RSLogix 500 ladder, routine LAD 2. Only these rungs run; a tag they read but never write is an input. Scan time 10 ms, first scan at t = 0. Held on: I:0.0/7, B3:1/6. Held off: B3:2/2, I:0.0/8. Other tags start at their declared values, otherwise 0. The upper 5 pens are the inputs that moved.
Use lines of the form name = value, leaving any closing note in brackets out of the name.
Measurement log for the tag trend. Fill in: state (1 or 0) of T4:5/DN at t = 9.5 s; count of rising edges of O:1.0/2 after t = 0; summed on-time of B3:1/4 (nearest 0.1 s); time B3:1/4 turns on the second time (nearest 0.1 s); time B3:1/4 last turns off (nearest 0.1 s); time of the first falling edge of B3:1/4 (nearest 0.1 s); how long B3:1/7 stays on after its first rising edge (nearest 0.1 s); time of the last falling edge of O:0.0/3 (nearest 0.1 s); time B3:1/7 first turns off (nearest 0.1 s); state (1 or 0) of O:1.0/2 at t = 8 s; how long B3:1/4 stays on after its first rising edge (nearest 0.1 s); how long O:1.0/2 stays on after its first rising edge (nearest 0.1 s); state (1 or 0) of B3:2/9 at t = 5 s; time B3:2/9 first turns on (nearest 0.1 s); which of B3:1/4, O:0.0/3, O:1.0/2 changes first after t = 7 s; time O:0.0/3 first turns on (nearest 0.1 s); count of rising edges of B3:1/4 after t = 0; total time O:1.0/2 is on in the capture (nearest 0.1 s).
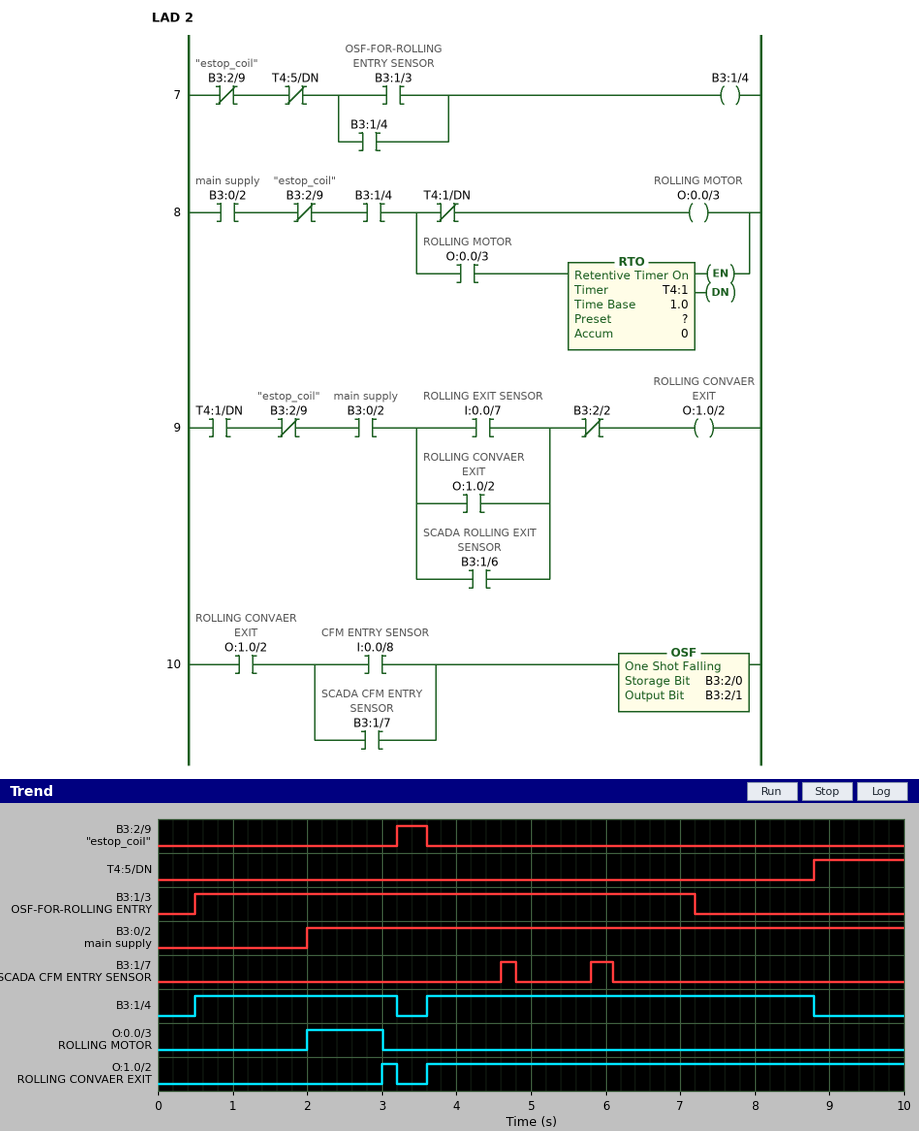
state (1 or 0) of T4:5/DN at t = 9.5 s = 1
count of rising edges of O:1.0/2 after t = 0 = 2
summed on-time of B3:1/4 = 7.9 s
time B3:1/4 turns on the second time = 3.6 s
time B3:1/4 last turns off = 8.8 s
time of the first falling edge of B3:1/4 = 3.2 s
how long B3:1/7 stays on after its first rising edge = 0.2 s
time of the last falling edge of O:0.0/3 = 3.0 s
time B3:1/7 first turns off = 4.8 s
state (1 or 0) of O:1.0/2 at t = 8 s = 1
how long B3:1/4 stays on after its first rising edge = 2.7 s
how long O:1.0/2 stays on after its first rising edge = 0.2 s
state (1 or 0) of B3:2/9 at t = 5 s = 0
time B3:2/9 first turns on = 3.2 s
which of B3:1/4, O:0.0/3, O:1.0/2 changes first after t = 7 s = B3:1/4
time O:0.0/3 first turns on = 2.0 s
count of rising edges of B3:1/4 after t = 0 = 2
total time O:1.0/2 is on in the capture = 6.6 s
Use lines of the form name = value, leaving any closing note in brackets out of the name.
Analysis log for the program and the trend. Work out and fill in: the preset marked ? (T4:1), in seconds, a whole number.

the preset marked ? (T4:1), in seconds, a whole number = 1 s
